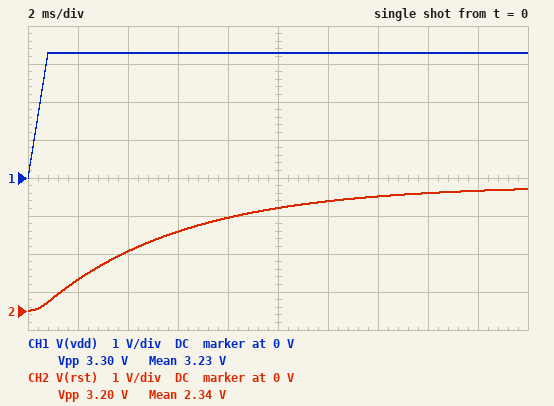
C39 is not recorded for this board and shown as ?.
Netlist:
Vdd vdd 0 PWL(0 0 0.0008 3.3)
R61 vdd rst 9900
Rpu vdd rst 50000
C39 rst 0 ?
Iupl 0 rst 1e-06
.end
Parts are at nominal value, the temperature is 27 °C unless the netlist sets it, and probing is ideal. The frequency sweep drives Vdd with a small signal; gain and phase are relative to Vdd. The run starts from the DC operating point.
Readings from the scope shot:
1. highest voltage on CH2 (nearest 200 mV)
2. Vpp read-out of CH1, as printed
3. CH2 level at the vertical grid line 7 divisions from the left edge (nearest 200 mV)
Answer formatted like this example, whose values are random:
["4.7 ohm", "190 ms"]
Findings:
["3.2 V", "3.30 V", "3.0 V"]
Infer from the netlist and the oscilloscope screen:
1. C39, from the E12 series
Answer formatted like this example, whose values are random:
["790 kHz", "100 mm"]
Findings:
["680 nF"]
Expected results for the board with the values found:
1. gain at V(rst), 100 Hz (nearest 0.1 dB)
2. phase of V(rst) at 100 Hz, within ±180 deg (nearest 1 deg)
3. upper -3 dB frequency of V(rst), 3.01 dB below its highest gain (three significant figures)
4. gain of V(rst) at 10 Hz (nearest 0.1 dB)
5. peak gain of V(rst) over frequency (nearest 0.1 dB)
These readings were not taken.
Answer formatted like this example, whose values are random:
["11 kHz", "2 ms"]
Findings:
["-11.3 dB", "-74 deg", "28.3 Hz", "-0.5 dB", "0 dB"]
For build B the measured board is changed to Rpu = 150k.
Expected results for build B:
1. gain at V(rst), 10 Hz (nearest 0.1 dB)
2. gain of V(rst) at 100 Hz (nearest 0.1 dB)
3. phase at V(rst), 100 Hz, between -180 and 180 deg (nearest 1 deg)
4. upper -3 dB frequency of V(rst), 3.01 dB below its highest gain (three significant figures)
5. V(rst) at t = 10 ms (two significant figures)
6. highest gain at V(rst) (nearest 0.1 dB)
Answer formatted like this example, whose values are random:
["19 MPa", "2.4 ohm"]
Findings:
["-0.6 dB", "-12.2 dB", "-76 deg", "25.2 Hz", "2.6 V", "0 dB"]
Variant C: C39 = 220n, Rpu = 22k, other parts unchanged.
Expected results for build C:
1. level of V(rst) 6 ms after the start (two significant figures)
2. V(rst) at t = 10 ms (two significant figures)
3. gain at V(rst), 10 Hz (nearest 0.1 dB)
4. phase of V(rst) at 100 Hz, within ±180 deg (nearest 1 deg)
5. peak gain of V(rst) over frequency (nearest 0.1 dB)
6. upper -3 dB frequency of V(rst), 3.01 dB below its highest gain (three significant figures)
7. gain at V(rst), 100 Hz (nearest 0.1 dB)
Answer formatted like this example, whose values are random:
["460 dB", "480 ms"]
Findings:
["3.2 V", "3.3 V", "0 dB", "-43 deg", "0 dB", "106 Hz", "-2.8 dB"]
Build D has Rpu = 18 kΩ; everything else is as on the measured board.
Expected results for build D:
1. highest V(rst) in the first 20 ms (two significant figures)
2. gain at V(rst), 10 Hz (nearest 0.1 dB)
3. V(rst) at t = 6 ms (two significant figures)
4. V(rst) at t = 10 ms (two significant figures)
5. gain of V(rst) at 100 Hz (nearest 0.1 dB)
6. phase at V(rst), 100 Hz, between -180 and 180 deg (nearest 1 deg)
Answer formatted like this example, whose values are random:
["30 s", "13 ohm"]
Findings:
["3.3 V", "-0.3 dB", "2.4 V", "2.9 V", "-9.3 dB", "-70 deg"]
